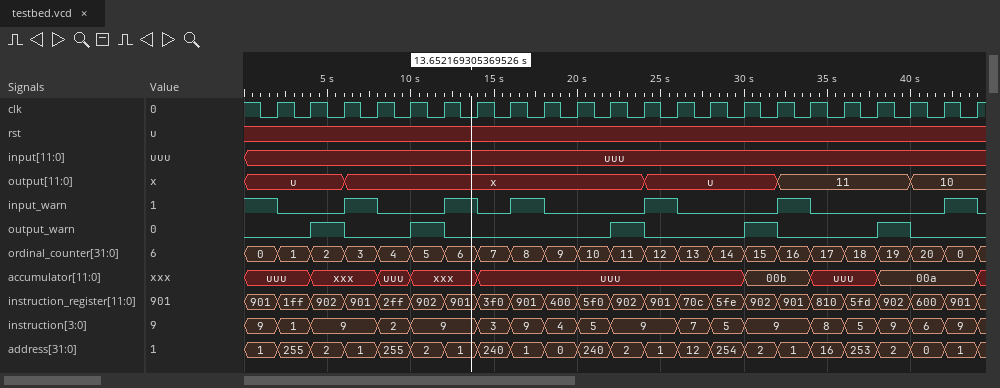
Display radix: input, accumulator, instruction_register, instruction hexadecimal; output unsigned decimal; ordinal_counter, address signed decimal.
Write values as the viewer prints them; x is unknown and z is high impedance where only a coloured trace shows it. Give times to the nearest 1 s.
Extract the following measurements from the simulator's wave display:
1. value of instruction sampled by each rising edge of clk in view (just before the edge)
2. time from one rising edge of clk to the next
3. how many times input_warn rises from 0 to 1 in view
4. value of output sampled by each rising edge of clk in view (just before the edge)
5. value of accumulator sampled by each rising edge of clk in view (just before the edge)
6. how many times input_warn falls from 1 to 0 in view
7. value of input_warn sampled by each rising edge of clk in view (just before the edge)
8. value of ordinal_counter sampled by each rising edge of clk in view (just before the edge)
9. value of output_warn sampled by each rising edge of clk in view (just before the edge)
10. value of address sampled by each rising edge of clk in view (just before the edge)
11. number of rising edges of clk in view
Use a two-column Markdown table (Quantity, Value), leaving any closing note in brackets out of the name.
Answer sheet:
| Quantity | Value |
|---|---|
| value of instruction sampled by each rising edge of clk in view | 9, 1, 9, 9, 2, 9, 9, 3, 9, 4, 5, 9, 9, 7, 5, 9, 9, 8, 5, 9, 6, 9 |
| time from one rising edge of clk to the next | 2 s |
| how many times input_warn rises from 0 to 1 in view | 6 |
| value of output sampled by each rising edge of clk in view | u, u, u, x, x, x, x, x, x, x, x, x, u, u, u, u, 11, 11, 11, 11, 10, 10 |
| value of accumulator sampled by each rising edge of clk in view | uuu, uuu, xxx, xxx, uuu, xxx, xxx, uuu, uuu, uuu, uuu, uuu, uuu, uuu, uuu, 00b, 00b, uuu, uuu, 00a, 00a, 00a |
| how many times input_warn falls from 1 to 0 in view | 7 |
| value of input_warn sampled by each rising edge of clk in view | 1 0 0 1 0 0 1 0 1 0 0 0 1 0 0 0 1 0 0 0 0 1 |
| value of ordinal_counter sampled by each rising edge of clk in view | 0, 1, 2, 3, 4, 5, 6, 7, 8, 9, 10, 11, 12, 13, 14, 15, 16, 17, 18, 19, 20, 0 |
| value of output_warn sampled by each rising edge of clk in view | 0 0 1 0 0 1 0 0 0 0 0 1 0 0 0 1 0 0 0 1 0 0 |
| value of address sampled by each rising edge of clk in view | 1, 255, 2, 1, 255, 2, 1, 240, 1, 0, 240, 2, 1, 12, 254, 2, 1, 16, 253, 2, 0, 1 |
| number of rising edges of clk in view | 22 |
